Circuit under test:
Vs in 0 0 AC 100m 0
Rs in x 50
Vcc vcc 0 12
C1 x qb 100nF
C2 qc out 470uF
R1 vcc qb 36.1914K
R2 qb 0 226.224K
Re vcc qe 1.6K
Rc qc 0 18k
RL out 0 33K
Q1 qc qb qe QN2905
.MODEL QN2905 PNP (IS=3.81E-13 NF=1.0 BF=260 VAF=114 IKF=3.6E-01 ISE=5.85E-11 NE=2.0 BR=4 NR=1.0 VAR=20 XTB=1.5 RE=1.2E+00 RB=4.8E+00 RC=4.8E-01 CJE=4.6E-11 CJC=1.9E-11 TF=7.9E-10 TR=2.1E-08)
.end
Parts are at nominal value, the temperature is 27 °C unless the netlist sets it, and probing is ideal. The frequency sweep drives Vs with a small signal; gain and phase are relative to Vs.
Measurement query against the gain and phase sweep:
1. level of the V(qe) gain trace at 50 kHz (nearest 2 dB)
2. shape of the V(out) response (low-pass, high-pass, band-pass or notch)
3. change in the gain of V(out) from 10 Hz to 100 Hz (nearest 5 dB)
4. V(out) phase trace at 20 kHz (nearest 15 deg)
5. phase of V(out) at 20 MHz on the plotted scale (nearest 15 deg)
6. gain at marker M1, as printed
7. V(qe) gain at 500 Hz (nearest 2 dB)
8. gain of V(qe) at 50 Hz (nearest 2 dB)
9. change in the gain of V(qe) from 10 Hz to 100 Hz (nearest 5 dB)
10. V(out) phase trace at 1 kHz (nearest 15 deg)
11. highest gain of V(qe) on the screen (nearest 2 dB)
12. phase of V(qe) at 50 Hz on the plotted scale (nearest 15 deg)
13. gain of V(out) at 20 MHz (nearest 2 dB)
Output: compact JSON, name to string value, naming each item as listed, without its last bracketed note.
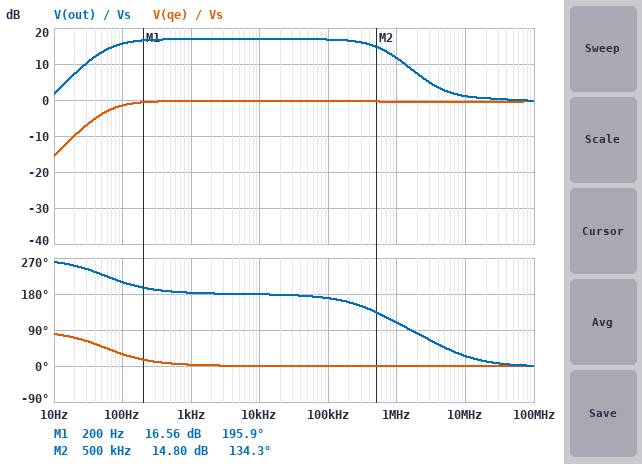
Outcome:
{"level of the V(qe) gain trace at 50 kHz": "0 dB", "shape of the V(out) response": "band-pass", "change in the gain of V(out) from 10 Hz to 100 Hz": "15 dB", "V(out) phase trace at 20 kHz": "180 deg", "phase of V(out) at 20 MHz on the plotted scale": "15 deg", "gain at marker M1, as printed": "16.56 dB", "V(qe) gain at 500 Hz": "0 dB", "gain of V(qe) at 50 Hz": "-4 dB", "change in the gain of V(qe) from 10 Hz to 100 Hz": "15 dB", "V(out) phase trace at 1 kHz": "180 deg", "highest gain of V(qe) on the screen": "0 dB", "phase of V(qe) at 50 Hz on the plotted scale": "45 deg", "gain of V(out) at 20 MHz": "0 dB"}
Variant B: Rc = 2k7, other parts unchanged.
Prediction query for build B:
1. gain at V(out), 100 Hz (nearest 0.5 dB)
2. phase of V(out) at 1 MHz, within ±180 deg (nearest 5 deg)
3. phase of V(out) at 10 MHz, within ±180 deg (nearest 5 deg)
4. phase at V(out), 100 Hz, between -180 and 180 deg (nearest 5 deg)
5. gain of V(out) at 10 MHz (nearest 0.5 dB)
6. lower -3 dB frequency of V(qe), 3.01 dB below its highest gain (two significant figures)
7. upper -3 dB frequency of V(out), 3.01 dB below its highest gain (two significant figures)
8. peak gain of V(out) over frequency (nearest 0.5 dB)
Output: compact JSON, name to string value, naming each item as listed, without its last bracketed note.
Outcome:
{"gain at V(out), 100 Hz": "2.5 dB", "phase of V(out) at 1 MHz, within ±180 deg": "165 deg", "phase of V(out) at 10 MHz, within ±180 deg": "80 deg", "phase at V(out), 100 Hz, between -180 and 180 deg": "-150 deg", "gain of V(out) at 10 MHz": "2.0 dB", "lower -3 dB frequency of V(qe), 3.01 dB below its highest gain": "56 Hz", "upper -3 dB frequency of V(out), 3.01 dB below its highest gain": "43 MHz", "peak gain of V(out) over frequency": "3.5 dB"}
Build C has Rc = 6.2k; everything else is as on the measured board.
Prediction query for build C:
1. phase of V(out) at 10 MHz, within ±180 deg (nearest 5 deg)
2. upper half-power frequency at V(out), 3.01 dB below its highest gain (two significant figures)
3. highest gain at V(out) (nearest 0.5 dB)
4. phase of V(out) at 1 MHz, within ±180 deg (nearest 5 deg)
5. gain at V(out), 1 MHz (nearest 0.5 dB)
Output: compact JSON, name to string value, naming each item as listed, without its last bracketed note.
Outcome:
{"phase of V(out) at 10 MHz, within ±180 deg": "60 deg", "upper half-power frequency at V(out), 3.01 dB below its highest gain": "3.8 MHz", "highest gain at V(out)": "10.0 dB", "phase of V(out) at 1 MHz, within ±180 deg": "155 deg", "gain at V(out), 1 MHz": "9.5 dB"}
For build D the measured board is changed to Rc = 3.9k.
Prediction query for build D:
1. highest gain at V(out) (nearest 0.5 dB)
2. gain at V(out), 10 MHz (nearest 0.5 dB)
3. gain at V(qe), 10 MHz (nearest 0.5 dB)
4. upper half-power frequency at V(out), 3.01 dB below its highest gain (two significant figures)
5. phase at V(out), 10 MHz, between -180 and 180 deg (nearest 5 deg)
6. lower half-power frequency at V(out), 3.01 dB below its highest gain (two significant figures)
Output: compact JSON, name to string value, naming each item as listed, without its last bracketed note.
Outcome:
{"highest gain at V(out)": "6.5 dB", "gain at V(out), 10 MHz": "3.0 dB", "gain at V(qe), 10 MHz": "-0.5 dB", "upper half-power frequency at V(out), 3.01 dB below its highest gain": "8.0 MHz", "phase at V(out), 10 MHz, between -180 and 180 deg": "70 deg", "lower half-power frequency at V(out), 3.01 dB below its highest gain": "56 Hz"}
